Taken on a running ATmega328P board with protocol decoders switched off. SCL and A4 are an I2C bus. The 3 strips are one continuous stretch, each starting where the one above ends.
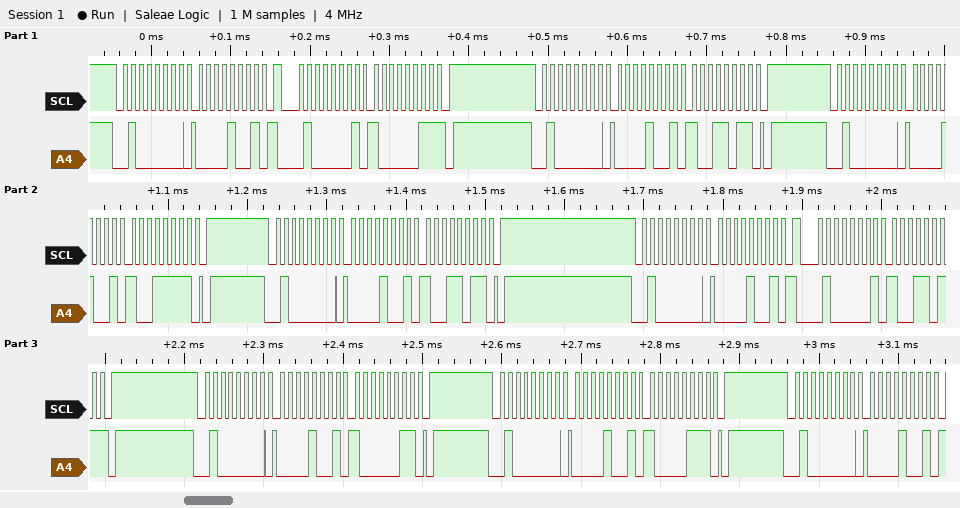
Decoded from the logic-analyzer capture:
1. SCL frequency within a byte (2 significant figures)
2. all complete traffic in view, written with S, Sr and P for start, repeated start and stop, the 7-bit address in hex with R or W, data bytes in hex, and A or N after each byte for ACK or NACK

100 kHz
S 20W A 09 A Sr 20R A 83 N P S 20W A 09 A 9B A P S 20W A 09 A 9F A P S 20W A 09 A 9B A P S 20W A 09 A Sr 20R A 9B N P S 20W A 09 A 83 A P S 20W A 09 A 87 A P S 20W A 09 A
